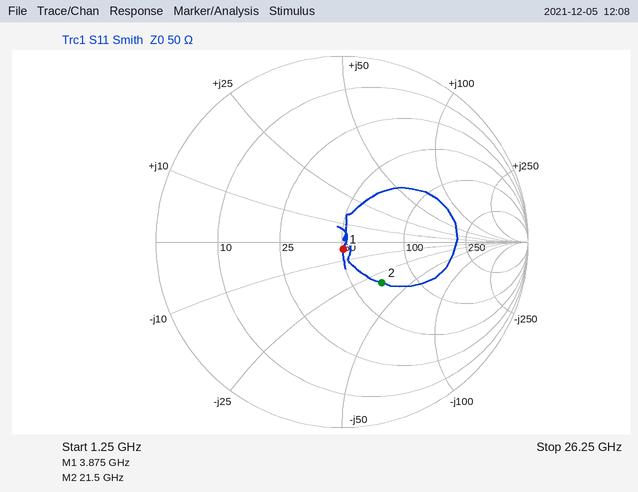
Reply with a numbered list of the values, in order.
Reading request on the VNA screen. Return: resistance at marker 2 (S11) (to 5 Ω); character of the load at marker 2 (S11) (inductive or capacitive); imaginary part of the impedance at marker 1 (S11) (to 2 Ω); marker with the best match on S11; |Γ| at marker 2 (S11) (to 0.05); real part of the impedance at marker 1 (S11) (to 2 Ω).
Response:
1. 70 Ω
2. capacitive
3. -4 Ω
4. marker 1
5. 0.30
6. 50 Ω
